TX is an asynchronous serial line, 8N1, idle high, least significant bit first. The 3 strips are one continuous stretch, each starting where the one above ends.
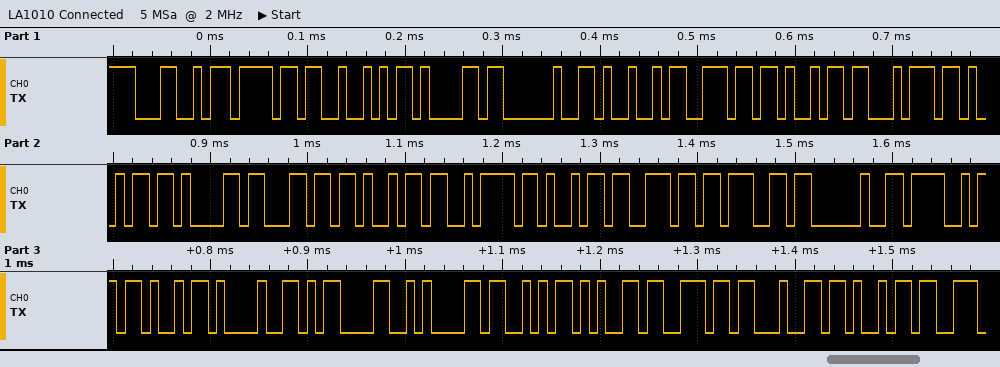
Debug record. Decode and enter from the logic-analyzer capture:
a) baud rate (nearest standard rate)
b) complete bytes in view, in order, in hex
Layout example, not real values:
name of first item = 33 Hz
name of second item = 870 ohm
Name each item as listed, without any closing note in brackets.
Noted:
baud rate = 115200 baud
complete bytes in view, in order, in hex = 0x4C 0x6F 0x52 0x61 0x20 0x49 0x6E 0x69 0x74 0x69 0x61 0x6C 0x69 0x7A 0x69 0x6E 0x67 0x20 0x4F 0x4B 0x21 0x0D 0x0A 0x53 0x65 0x6E 0x64 0x69
